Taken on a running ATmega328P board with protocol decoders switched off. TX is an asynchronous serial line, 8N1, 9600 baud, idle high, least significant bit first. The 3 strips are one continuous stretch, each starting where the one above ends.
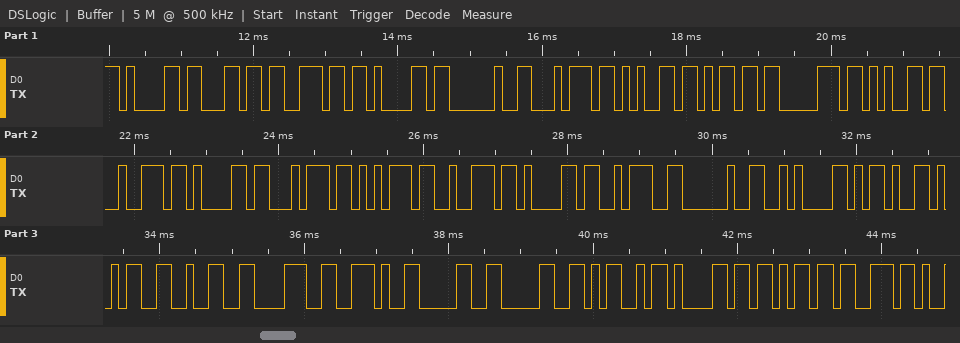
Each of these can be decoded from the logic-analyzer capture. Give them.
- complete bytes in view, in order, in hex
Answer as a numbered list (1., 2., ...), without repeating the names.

1. 61 6C 6E 61 20 74 65 6D 70 65 72 61 74 75 72 61 3A 20 0A 2D 35 32 38 2E 30 30 4D 61 6B 73
